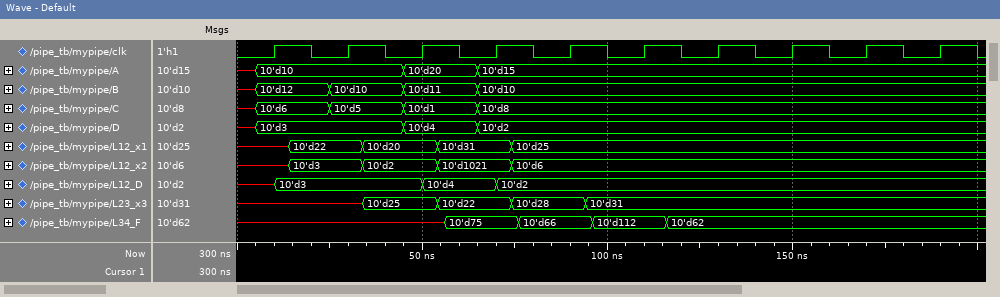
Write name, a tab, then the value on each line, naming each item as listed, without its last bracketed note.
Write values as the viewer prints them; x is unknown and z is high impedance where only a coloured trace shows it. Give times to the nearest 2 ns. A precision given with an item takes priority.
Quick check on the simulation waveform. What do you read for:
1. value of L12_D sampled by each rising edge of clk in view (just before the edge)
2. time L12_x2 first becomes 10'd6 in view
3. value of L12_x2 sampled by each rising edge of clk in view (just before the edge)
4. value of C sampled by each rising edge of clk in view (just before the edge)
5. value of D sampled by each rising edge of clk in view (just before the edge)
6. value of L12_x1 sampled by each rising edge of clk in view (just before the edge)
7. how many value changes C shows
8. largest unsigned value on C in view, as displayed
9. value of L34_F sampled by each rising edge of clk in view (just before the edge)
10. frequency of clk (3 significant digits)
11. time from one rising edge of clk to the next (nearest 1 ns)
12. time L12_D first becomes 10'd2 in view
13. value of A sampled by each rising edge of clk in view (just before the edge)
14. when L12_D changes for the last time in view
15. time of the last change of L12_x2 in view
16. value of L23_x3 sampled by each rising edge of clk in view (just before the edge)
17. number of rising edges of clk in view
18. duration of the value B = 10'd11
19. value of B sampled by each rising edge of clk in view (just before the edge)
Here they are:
value of L12_D sampled by each rising edge of clk in view	x, 10'd3, 10'd3, 10'd4, 10'd2, 10'd2, 10'd2, 10'd2, 10'd2, 10'd2
time L12_x2 first becomes 10'd6 in view	74 ns
value of L12_x2 sampled by each rising edge of clk in view	x, 10'd3, 10'd2, 10'd1021, 10'd6, 10'd6, 10'd6, 10'd6, 10'd6, 10'd6
value of C sampled by each rising edge of clk in view	10'd6, 10'd5, 10'd1, 10'd8, 10'd8, 10'd8, 10'd8, 10'd8, 10'd8, 10'd8
value of D sampled by each rising edge of clk in view	10'd3, 10'd3, 10'd4, 10'd2, 10'd2, 10'd2, 10'd2, 10'd2, 10'd2, 10'd2
value of L12_x1 sampled by each rising edge of clk in view	x, 10'd22, 10'd20, 10'd31, 10'd25, 10'd25, 10'd25, 10'd25, 10'd25, 10'd25
how many value changes C shows	4
largest unsigned value on C in view, as displayed	10'd8
value of L34_F sampled by each rising edge of clk in view	x, x, x, 10'd75, 10'd66, 10'd112, 10'd62, 10'd62, 10'd62, 10'd62
frequency of clk	50.0 MHz
time from one rising edge of clk to the next	20 ns
time L12_D first becomes 10'd2 in view	70 ns
value of A sampled by each rising edge of clk in view	10'd10, 10'd10, 10'd20, 10'd15, 10'd15, 10'd15, 10'd15, 10'd15, 10'd15, 10'd15
when L12_D changes for the last time in view	70 ns
time of the last change of L12_x2 in view	74 ns
value of L23_x3 sampled by each rising edge of clk in view	x, x, 10'd25, 10'd22, 10'd28, 10'd31, 10'd31, 10'd31, 10'd31, 10'd31
number of rising edges of clk in view	10
duration of the value B = 10'd11	20 ns
value of B sampled by each rising edge of clk in view	10'd12, 10'd10, 10'd11, 10'd10, 10'd10, 10'd10, 10'd10, 10'd10, 10'd10, 10'd10
